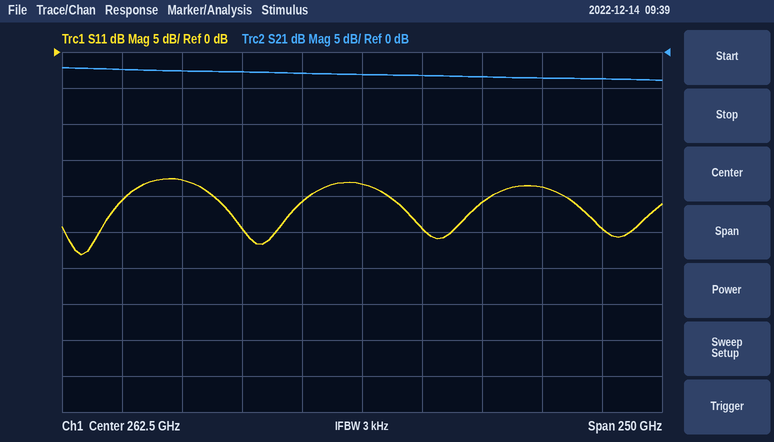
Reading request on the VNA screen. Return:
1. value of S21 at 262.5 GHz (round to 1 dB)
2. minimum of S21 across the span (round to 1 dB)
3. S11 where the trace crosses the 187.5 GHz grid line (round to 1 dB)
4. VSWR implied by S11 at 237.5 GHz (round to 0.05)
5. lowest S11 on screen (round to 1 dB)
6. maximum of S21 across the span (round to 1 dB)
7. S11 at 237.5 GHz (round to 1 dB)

-3 dB
-4 dB
-18 dB
1.20
-28 dB
-2 dB
-21 dB
